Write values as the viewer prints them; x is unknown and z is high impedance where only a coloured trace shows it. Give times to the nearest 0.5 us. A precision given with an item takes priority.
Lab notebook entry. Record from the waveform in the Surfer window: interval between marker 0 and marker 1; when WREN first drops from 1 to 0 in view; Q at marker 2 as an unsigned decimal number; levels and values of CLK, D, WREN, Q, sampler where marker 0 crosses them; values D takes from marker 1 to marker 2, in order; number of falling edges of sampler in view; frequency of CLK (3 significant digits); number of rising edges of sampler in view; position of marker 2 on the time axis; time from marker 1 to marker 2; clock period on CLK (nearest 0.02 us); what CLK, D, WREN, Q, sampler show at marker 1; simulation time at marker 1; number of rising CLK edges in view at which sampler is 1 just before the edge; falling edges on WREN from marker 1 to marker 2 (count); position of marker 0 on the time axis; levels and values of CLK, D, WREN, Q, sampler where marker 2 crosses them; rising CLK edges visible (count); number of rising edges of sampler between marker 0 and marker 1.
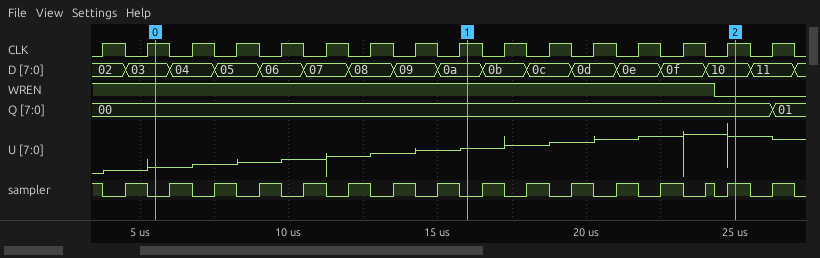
10.5 us
24.5 us
0
CLK=1, D=03, WREN=1, Q=00, sampler=0
0a, 0b, 0c, 0d, 0e, 0f, 10
17
667 kHz
16
25 us
9 us
1.5 us
CLK=1, D=0a, WREN=1, Q=00, sampler=0
16 us
14
1
5.5 us
CLK=1, D=10, WREN=0, Q=00, sampler=1
16
7
